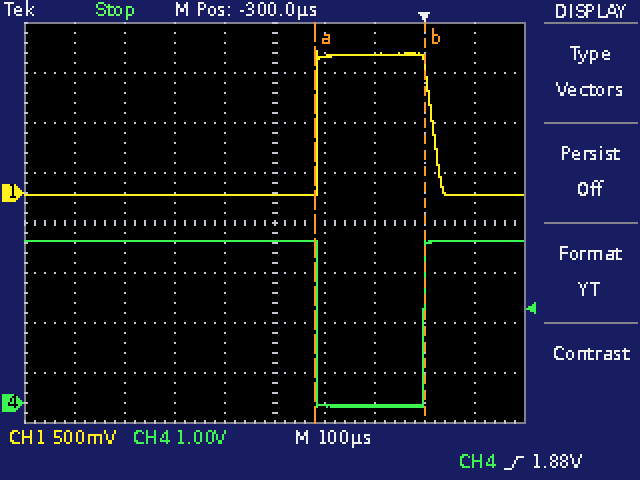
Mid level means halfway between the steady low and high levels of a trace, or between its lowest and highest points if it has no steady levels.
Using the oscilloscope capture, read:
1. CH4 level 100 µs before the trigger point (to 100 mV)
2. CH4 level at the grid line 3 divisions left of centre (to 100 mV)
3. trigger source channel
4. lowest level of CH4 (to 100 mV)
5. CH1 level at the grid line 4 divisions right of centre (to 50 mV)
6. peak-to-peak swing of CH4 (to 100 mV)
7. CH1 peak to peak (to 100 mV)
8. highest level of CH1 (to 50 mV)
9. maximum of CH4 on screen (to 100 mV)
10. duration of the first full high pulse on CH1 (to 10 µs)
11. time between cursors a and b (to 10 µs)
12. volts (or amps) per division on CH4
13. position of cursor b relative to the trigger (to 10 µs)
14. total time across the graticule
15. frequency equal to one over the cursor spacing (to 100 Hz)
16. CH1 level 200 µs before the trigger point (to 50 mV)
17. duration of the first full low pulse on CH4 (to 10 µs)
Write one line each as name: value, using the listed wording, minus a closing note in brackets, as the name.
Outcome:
CH4 level 100 µs before the trigger point: -100 mV
CH4 level at the grid line 3 divisions left of centre: 3.2 V
trigger source channel: CH4
lowest level of CH4: -100 mV
CH1 level at the grid line 4 divisions right of centre: 0 mV
peak-to-peak swing of CH4: 3.3 V
CH1 peak to peak: 1.40 V
highest level of CH1: 1.40 V
maximum of CH4 on screen: 3.2 V
duration of the first full high pulse on CH1: 230 µs
time between cursors a and b: 220 µs
volts (or amps) per division on CH4: 1 V
position of cursor b relative to the trigger: 0 µs
total time across the graticule: 1 ms
frequency equal to one over the cursor spacing: 4.5 kHz
CH1 level 200 µs before the trigger point: 1.35 V
duration of the first full low pulse on CH4: 210 µs
